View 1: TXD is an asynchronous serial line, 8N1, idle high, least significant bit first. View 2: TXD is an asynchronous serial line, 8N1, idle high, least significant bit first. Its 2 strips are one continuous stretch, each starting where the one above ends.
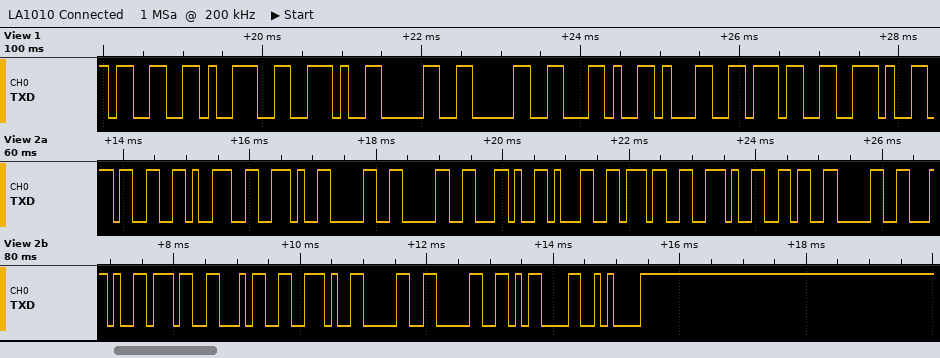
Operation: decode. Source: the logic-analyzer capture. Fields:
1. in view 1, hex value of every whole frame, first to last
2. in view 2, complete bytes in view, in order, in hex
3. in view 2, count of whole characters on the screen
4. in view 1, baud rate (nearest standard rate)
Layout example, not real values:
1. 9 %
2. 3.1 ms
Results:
1. 0x33 0x39 0x2E 0x30 0x30 0x2C 0x31 0x37 0x2E
2. 33 39 2E 30 30 2C 31 37 2E 36 30 2C 37 34 2E 30 30 0D 0A
3. 19
4. 9600 baud
